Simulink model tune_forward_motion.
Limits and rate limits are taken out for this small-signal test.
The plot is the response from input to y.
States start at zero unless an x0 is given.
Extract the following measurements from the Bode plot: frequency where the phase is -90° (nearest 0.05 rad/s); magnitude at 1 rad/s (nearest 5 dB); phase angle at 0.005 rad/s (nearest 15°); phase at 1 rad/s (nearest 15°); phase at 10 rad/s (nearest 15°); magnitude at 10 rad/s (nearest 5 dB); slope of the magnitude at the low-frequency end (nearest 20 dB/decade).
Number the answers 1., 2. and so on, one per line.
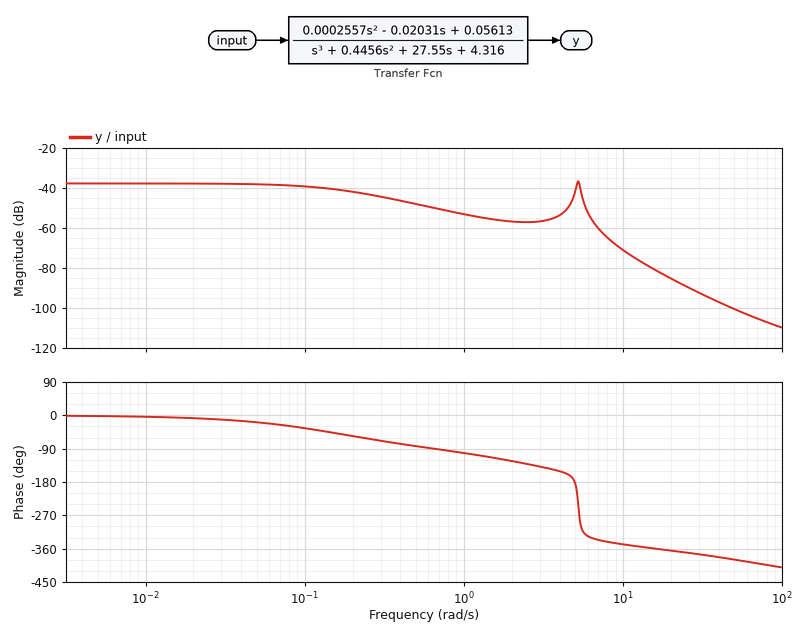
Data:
1. 0.65 rad/s
2. -55 dB
3. 0°
4. -105°
5. -345°
6. -70 dB
7. 0 dB/decade
